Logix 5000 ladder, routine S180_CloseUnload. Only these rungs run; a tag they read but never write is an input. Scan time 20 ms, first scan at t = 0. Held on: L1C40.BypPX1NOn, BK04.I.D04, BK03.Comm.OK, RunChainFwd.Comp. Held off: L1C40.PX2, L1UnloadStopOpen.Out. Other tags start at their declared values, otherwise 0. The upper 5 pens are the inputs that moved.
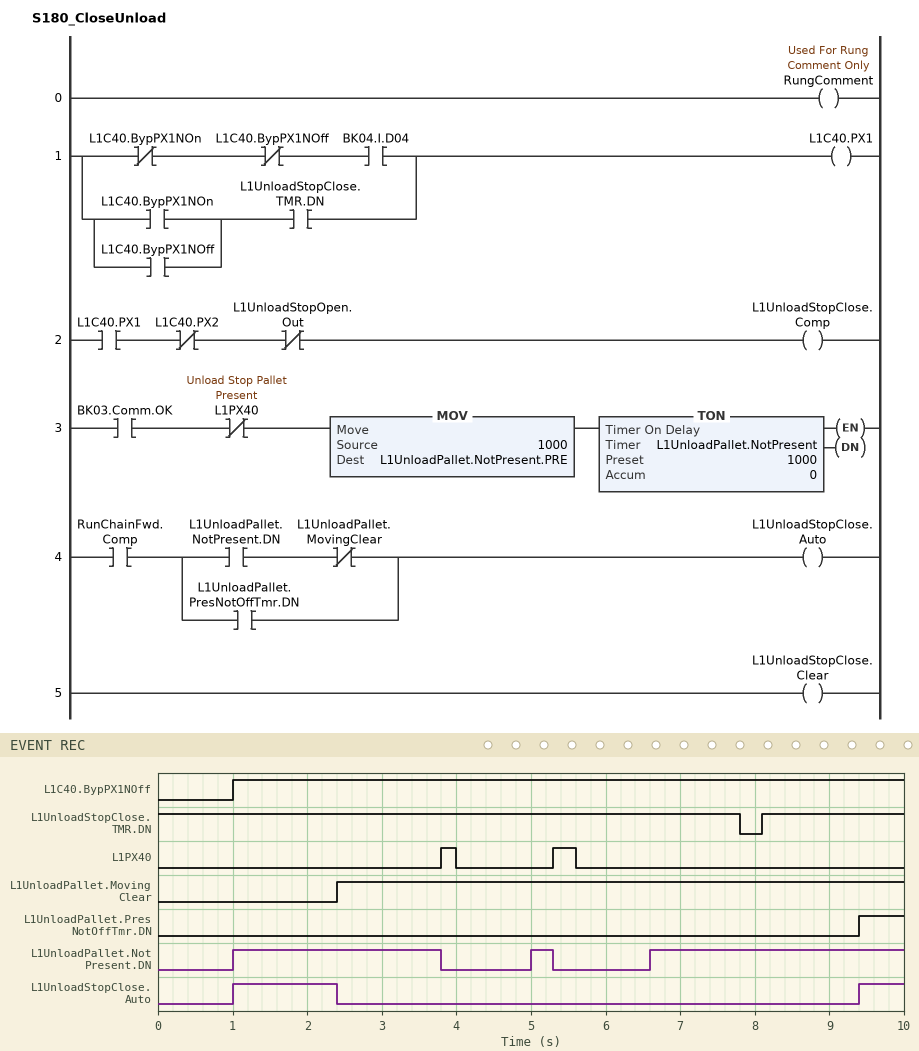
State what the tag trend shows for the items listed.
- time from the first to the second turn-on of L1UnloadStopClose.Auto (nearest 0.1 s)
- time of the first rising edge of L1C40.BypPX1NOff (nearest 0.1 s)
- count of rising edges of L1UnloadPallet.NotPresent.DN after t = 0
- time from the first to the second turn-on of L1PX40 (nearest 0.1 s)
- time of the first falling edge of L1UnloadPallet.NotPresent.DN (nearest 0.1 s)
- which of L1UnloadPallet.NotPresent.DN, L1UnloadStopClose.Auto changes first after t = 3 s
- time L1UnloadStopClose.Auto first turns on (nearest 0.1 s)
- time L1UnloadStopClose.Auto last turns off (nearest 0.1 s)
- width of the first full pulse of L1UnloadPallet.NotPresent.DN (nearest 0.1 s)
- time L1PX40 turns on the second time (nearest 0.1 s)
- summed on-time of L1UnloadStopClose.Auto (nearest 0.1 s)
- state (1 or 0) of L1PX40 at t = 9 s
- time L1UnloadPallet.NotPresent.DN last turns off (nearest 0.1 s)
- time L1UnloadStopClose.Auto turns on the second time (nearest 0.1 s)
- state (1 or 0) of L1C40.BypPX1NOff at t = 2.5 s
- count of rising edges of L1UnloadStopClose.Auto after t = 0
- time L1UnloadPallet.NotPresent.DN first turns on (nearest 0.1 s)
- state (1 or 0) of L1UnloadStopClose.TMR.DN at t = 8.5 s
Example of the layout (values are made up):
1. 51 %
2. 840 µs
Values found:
1. 8.4 s
2. 1.0 s
3. 3
4. 1.5 s
5. 3.8 s
6. L1UnloadPallet.NotPresent.DN
7. 1.0 s
8. 2.4 s
9. 2.8 s
10. 5.3 s
11. 2.0 s
12. 0
13. 5.3 s
14. 9.4 s
15. 1
16. 2
17. 1.0 s
18. 1
